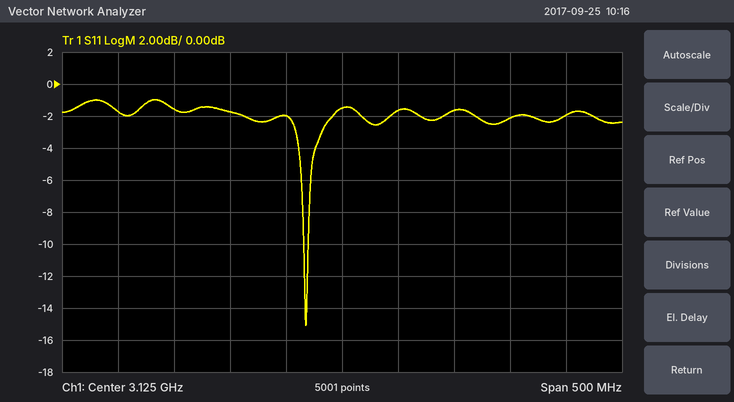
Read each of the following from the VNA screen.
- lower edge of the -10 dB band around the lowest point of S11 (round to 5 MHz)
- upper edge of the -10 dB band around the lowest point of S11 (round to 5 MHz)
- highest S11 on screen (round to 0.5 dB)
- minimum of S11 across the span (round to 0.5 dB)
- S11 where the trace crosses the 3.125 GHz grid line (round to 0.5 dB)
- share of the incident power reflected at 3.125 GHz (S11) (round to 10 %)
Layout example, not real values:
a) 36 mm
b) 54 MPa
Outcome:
a) 3.090 GHz
b) 3.095 GHz
c) -1.0 dB
d) -15.0 dB
e) -1.5 dB
f) 70 %
